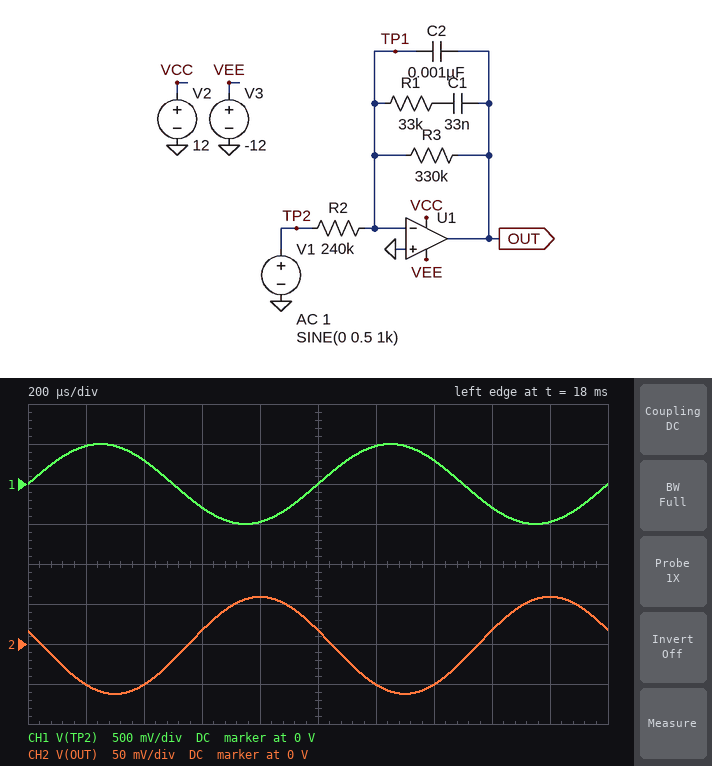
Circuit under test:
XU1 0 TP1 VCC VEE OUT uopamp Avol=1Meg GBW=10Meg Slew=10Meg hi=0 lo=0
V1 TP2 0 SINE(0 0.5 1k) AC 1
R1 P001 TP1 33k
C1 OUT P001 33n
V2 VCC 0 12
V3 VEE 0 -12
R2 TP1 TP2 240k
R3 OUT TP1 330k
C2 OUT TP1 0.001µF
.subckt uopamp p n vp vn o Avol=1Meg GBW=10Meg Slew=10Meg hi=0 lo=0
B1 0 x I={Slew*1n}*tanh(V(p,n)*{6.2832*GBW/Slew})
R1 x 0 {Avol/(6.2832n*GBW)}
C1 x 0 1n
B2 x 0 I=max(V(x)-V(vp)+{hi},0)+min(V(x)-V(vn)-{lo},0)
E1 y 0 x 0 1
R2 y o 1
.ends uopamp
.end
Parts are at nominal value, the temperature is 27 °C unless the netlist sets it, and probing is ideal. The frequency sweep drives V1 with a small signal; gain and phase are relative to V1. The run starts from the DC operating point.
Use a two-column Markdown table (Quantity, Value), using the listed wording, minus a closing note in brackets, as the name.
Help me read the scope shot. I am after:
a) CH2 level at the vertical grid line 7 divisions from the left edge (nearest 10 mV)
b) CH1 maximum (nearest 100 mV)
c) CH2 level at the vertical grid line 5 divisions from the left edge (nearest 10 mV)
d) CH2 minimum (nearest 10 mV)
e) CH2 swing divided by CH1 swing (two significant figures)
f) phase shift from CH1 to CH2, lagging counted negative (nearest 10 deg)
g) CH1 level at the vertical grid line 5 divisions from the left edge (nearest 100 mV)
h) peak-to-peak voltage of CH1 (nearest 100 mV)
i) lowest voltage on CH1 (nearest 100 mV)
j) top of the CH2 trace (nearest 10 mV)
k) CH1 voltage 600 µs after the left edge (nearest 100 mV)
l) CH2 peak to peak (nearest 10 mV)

| Quantity | Value |
|---|---|
| CH2 level at the vertical grid line 7 divisions from the left edge | -50 mV |
| CH1 maximum | 500 mV |
| CH2 level at the vertical grid line 5 divisions from the left edge | 20 mV |
| CH2 minimum | -60 mV |
| CH2 swing divided by CH1 swing | 0.12 |
| phase shift from CH1 to CH2, lagging counted negative | 160 deg |
| CH1 level at the vertical grid line 5 divisions from the left edge | 0 V |
| peak-to-peak voltage of CH1 | 1.0 V |
| lowest voltage on CH1 | -500 mV |
| top of the CH2 trace | 60 mV |
| CH1 voltage 600 µs after the left edge | -300 mV |
| CH2 peak to peak | 120 mV |
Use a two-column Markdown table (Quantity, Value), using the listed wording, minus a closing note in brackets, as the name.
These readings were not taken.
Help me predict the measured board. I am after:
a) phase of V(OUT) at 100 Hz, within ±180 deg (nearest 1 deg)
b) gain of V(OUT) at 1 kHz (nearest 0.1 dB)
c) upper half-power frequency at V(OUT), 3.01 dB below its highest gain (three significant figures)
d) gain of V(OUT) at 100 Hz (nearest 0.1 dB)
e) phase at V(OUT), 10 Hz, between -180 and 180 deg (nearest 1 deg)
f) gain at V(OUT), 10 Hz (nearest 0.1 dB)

| Quantity | Value |
|---|---|
| phase of V(OUT) at 100 Hz, within ±180 deg | 131 deg |
| gain of V(OUT) at 1 kHz | -18.3 dB |
| upper half-power frequency at V(OUT), 3.01 dB below its highest gain | 13.1 Hz |
| gain of V(OUT) at 100 Hz | -13.4 dB |
| phase at V(OUT), 10 Hz, between -180 and 180 deg | 146 deg |
| gain at V(OUT), 10 Hz | 0.8 dB |
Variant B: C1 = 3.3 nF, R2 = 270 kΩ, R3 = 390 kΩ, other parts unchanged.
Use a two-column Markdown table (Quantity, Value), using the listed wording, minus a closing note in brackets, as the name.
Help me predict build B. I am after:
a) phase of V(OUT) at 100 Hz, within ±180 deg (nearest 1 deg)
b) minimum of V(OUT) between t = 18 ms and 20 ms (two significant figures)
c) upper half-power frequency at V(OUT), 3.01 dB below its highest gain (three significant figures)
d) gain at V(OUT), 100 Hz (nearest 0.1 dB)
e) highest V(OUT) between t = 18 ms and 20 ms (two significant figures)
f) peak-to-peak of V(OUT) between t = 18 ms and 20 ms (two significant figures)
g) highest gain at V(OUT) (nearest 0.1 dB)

| Quantity | Value |
|---|---|
| phase of V(OUT) at 100 Hz, within ±180 deg | 135 deg |
| minimum of V(OUT) between t = 18 ms and 20 ms | -78 mV |
| upper half-power frequency at V(OUT), 3.01 dB below its highest gain | 90.7 Hz |
| gain at V(OUT), 100 Hz | -0.3 dB |
| highest V(OUT) between t = 18 ms and 20 ms | 78 mV |
| peak-to-peak of V(OUT) between t = 18 ms and 20 ms | 160 mV |
| highest gain at V(OUT) | 3.2 dB |
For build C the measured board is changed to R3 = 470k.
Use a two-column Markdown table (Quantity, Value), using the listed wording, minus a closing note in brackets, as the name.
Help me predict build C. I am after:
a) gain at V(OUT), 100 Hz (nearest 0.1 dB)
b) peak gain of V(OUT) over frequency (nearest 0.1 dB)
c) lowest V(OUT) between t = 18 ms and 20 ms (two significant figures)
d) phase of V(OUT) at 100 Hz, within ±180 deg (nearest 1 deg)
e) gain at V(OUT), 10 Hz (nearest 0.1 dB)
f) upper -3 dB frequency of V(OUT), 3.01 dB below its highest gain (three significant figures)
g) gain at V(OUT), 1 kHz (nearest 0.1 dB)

| Quantity | Value |
|---|---|
| gain at V(OUT), 100 Hz | -13.1 dB |
| peak gain of V(OUT) over frequency | 5.8 dB |
| lowest V(OUT) between t = 18 ms and 20 ms | -65 mV |
| phase of V(OUT) at 100 Hz, within ±180 deg | 129 deg |
| gain at V(OUT), 10 Hz | 2.5 dB |
| upper -3 dB frequency of V(OUT), 3.01 dB below its highest gain | 9.38 Hz |
| gain at V(OUT), 1 kHz | -18.1 dB |
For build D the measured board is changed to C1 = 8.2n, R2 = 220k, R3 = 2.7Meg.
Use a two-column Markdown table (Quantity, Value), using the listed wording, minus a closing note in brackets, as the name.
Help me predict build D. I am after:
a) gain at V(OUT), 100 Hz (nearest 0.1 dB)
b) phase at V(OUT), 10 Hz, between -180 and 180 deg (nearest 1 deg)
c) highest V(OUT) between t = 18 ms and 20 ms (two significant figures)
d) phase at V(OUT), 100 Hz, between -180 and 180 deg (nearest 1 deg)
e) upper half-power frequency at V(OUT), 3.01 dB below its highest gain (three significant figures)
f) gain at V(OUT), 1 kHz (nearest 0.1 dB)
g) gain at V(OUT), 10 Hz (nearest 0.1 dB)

| Quantity | Value |
|---|---|
| gain at V(OUT), 100 Hz | -2.1 dB |
| phase at V(OUT), 10 Hz, between -180 and 180 deg | 123 deg |
| highest V(OUT) between t = 18 ms and 20 ms | 58 mV |
| phase at V(OUT), 100 Hz, between -180 and 180 deg | 102 deg |
| upper half-power frequency at V(OUT), 3.01 dB below its highest gain | 6.35 Hz |
| gain at V(OUT), 1 kHz | -16.4 dB |
| gain at V(OUT), 10 Hz | 16.4 dB |
